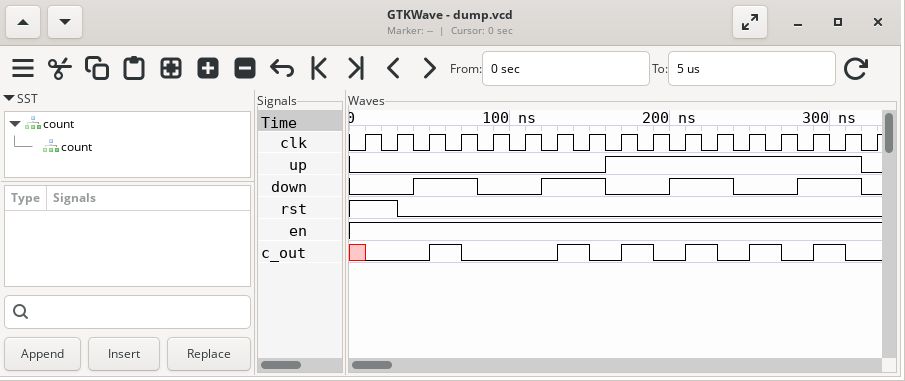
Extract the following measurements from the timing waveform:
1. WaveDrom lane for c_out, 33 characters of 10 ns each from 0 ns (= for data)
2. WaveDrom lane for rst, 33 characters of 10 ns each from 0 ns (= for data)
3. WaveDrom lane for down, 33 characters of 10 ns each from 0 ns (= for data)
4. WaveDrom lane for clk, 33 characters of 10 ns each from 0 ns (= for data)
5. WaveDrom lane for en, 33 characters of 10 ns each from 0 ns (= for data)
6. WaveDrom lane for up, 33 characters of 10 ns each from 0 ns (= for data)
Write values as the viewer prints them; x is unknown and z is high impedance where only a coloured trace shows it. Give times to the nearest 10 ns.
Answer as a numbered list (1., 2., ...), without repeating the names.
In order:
1. {name: 'c_out', wave: 'x0...1.0.....1.0.1.0.1.0.1.0.1.0.'}
2. {name: 'rst', wave: '1..0.............................'}
3. {name: 'down', wave: '0...1...0...1...0...1...0...1...0'}
4. {name: 'clk', wave: '010101010101010101010101010101010'}
5. {name: 'en', wave: '1................................'}
6. {name: 'up', wave: '0...............1...............0'}
